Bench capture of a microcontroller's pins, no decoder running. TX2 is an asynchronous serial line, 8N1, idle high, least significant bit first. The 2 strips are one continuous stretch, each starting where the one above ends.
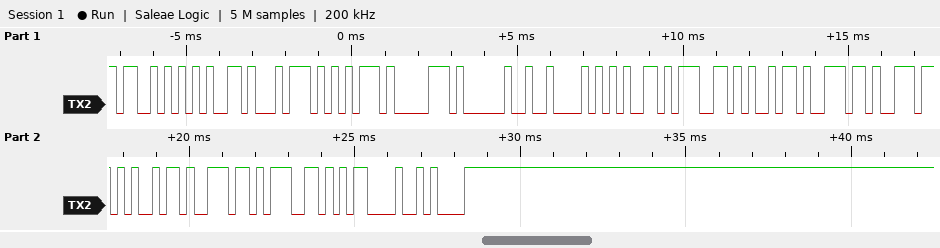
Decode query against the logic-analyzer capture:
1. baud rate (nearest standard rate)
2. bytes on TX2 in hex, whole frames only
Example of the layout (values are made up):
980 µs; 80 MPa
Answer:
4800 baud; 0x53 0x65 0x74 0x75 0x70 0x20 0x42 0x65 0x67 0x69 0x6E 0x6E 0x69 0x6E 0x67 0x0D 0x0A
